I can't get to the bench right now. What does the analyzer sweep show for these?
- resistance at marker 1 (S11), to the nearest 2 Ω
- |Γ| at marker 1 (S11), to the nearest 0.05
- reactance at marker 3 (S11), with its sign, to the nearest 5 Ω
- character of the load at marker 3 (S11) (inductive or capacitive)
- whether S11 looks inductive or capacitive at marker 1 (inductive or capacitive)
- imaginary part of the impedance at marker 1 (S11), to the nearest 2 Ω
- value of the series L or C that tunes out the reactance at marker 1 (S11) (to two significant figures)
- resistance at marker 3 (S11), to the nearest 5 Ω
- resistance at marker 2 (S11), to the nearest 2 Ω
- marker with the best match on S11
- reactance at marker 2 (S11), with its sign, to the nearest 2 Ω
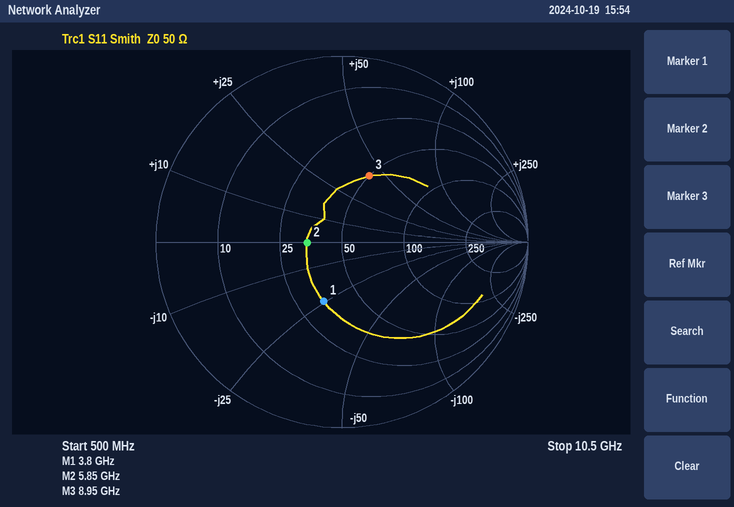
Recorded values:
34 Ω
0.35
+40 Ω
inductive
capacitive
-24 Ω
1.0 nH
50 Ω
34 Ω
marker 2
0 Ω
